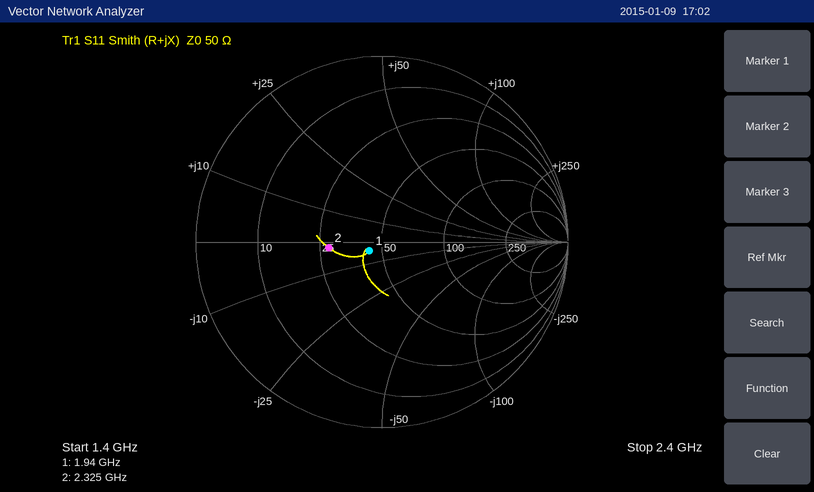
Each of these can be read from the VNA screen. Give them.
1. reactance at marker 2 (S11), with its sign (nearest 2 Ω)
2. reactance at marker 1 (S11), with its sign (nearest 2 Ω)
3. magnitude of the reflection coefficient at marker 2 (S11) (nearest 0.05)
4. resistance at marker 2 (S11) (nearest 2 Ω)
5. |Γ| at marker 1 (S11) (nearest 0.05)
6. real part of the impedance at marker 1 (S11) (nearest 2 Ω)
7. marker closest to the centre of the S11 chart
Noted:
-2 Ω
-4 Ω
0.30
28 Ω
0.10
44 Ω
marker 1
